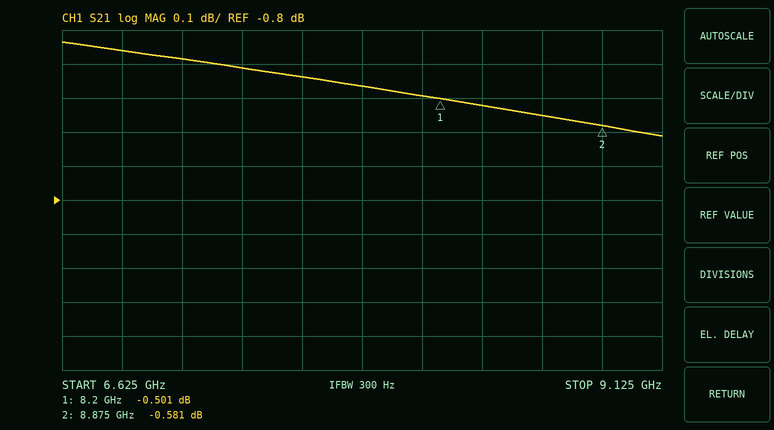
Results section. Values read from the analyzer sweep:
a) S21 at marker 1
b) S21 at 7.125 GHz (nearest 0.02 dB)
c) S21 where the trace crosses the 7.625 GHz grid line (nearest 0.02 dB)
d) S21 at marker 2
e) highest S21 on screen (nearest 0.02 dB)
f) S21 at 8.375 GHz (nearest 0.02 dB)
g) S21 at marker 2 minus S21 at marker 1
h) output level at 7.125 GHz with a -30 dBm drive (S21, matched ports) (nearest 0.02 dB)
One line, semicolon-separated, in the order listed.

-0.501 dB; -0.38 dB; -0.44 dB; -0.581 dB; -0.34 dB; -0.52 dB; -0.080 dB; -30.38 dBm
